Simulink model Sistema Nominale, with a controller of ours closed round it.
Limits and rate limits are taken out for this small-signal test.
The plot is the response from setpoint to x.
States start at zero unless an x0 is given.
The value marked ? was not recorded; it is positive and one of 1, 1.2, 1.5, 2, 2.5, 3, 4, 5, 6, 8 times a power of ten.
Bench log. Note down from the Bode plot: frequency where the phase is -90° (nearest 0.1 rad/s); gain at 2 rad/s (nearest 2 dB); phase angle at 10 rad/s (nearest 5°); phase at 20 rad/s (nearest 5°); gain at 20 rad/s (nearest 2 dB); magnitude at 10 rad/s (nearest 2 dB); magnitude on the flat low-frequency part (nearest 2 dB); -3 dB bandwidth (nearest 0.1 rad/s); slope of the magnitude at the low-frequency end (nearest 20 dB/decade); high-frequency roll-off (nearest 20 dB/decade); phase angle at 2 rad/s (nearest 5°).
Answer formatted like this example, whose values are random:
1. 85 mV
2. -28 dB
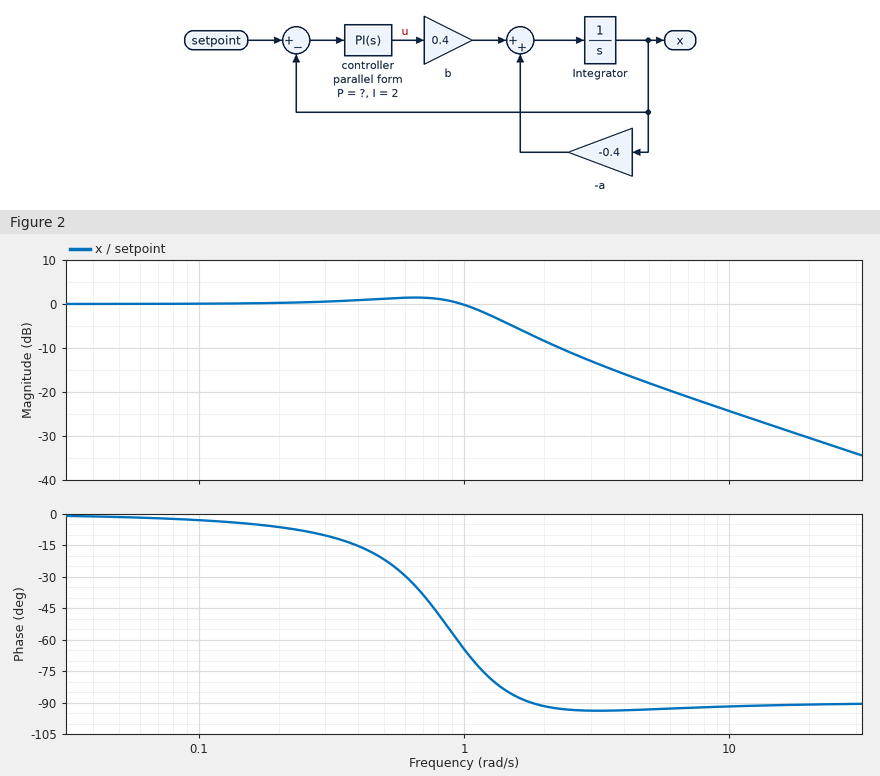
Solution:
1. 1.8 rad/s
2. -8 dB
3. -90°
4. -90°
5. -30 dB
6. -24 dB
7. 0 dB
8. 1.3 rad/s
9. 0 dB/decade
10. -20 dB/decade
11. -90°
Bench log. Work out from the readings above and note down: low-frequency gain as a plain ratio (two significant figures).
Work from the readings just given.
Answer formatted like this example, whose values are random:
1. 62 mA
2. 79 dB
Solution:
1. 1.0
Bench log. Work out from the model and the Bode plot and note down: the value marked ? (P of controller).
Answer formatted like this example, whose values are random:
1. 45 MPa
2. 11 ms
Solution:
1. 1.5
